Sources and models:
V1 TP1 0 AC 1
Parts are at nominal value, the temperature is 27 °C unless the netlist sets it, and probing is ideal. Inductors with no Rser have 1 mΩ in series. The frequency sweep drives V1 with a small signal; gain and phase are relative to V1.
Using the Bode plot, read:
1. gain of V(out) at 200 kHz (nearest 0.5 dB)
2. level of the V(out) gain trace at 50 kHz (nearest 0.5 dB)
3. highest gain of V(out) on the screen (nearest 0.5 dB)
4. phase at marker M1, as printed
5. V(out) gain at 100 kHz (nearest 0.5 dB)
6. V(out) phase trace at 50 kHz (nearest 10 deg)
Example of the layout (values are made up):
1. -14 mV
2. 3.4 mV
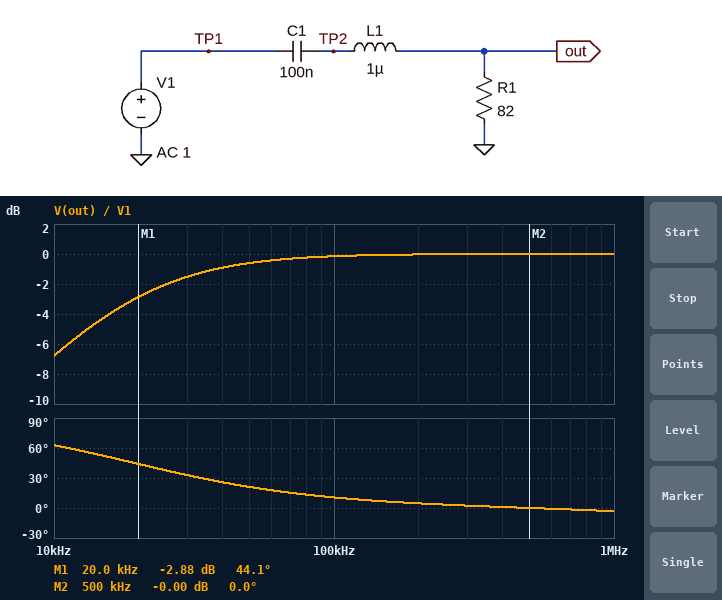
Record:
1. 0 dB
2. -0.5 dB
3. 0 dB
4. 44.1 deg
5. 0 dB
6. 20 deg
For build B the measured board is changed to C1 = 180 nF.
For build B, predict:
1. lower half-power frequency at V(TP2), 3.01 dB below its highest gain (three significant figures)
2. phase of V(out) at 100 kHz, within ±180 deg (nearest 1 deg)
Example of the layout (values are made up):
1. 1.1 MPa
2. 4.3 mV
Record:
1. 10.8 kHz
2. 6 deg
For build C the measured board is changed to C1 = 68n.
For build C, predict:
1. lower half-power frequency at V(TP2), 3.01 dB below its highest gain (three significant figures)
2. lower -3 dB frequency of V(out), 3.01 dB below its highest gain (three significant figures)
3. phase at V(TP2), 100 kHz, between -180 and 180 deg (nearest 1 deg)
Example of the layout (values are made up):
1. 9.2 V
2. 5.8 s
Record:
1. 28.6 kHz
2. 28.5 kHz
3. 16 deg
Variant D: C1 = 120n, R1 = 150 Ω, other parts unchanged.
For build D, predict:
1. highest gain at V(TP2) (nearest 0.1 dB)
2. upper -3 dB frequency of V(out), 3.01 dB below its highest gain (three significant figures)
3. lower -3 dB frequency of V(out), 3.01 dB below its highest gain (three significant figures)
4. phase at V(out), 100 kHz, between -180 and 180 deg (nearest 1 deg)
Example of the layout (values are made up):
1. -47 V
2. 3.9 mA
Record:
1. 0 dB
2. 23.9 MHz
3. 8.84 kHz
4. 5 deg
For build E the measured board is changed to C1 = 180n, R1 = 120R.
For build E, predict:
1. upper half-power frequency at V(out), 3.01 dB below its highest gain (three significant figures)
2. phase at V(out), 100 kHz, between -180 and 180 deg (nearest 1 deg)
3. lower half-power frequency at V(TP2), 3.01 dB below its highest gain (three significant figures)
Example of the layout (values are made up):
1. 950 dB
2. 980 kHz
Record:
1. 19.1 MHz
2. 4 deg
3. 7.37 kHz
